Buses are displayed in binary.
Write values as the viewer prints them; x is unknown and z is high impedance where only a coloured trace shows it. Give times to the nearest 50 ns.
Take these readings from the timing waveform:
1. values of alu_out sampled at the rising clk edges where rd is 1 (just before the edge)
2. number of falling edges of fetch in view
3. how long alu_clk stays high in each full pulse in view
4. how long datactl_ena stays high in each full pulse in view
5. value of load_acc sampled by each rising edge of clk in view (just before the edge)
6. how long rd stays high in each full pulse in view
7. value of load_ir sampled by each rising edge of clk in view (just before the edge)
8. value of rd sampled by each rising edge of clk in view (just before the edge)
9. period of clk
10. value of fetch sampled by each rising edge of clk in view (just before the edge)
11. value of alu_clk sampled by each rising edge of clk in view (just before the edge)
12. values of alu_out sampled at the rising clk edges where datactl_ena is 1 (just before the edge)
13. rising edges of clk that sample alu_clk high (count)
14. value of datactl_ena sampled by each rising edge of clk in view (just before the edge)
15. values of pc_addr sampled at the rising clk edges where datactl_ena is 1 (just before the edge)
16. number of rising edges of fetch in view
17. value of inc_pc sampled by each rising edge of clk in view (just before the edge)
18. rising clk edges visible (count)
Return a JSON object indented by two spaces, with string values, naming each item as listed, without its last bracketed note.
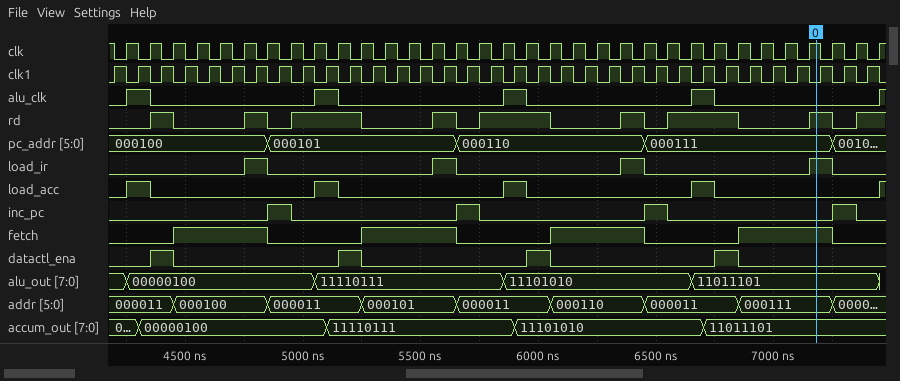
{
  "values of alu_out sampled at the rising clk edges where rd is 1": "00000100, 00000100, 00000100, 11110111, 11110111, 11110111, 11110111, 11101010, 11101010, 11101010, 11101010, 11011101, 11011101, 11011101, 11011101",
  "number of falling edges of fetch in view": "4",
  "how long alu_clk stays high in each full pulse in view": "100 ns, 100 ns, 100 ns, 100 ns",
  "how long datactl_ena stays high in each full pulse in view": "100 ns, 100 ns, 100 ns, 100 ns",
  "value of load_acc sampled by each rising edge of clk in view": "0 1 0 0 0 0 0 0 0 1 0 0 0 0 0 0 0 1 0 0 0 0 0 0 0 1 0 0 0 0 0 0 0",
  "how long rd stays high in each full pulse in view": "100 ns, 100 ns, 300 ns, 100 ns, 300 ns, 100 ns, 300 ns, 100 ns",
  "value of load_ir sampled by each rising edge of clk in view": "0 0 0 0 0 0 1 0 0 0 0 0 0 0 1 0 0 0 0 0 0 0 1 0 0 0 0 0 0 0 1 0 0",
  "value of rd sampled by each rising edge of clk in view": "0 0 1 0 0 0 1 0 1 1 1 0 0 0 1 0 1 1 1 0 0 0 1 0 1 1 1 0 0 0 1 0 1",
  "period of clk": "100 ns",
  "value of fetch sampled by each rising edge of clk in view": "0 0 0 1 1 1 1 0 0 0 0 1 1 1 1 0 0 0 0 1 1 1 1 0 0 0 0 1 1 1 1 0 0",
  "value of alu_clk sampled by each rising edge of clk in view": "0 1 0 0 0 0 0 0 0 1 0 0 0 0 0 0 0 1 0 0 0 0 0 0 0 1 0 0 0 0 0 0 0",
  "values of alu_out sampled at the rising clk edges where datactl_ena is 1": "00000100, 11110111, 11101010, 11011101",
  "rising edges of clk that sample alu_clk high": "4",
  "value of datactl_ena sampled by each rising edge of clk in view": "0 0 1 0 0 0 0 0 0 0 1 0 0 0 0 0 0 0 1 0 0 0 0 0 0 0 1 0 0 0 0 0 0",
  "values of pc_addr sampled at the rising clk edges where datactl_ena is 1": "000100, 000101, 000110, 000111",
  "number of rising edges of fetch in view": "4",
  "value of inc_pc sampled by each rising edge of clk in view": "0 0 0 0 0 0 0 1 0 0 0 0 0 0 0 1 0 0 0 0 0 0 0 1 0 0 0 0 0 0 0 1 0",
  "rising clk edges visible": "33"
}
